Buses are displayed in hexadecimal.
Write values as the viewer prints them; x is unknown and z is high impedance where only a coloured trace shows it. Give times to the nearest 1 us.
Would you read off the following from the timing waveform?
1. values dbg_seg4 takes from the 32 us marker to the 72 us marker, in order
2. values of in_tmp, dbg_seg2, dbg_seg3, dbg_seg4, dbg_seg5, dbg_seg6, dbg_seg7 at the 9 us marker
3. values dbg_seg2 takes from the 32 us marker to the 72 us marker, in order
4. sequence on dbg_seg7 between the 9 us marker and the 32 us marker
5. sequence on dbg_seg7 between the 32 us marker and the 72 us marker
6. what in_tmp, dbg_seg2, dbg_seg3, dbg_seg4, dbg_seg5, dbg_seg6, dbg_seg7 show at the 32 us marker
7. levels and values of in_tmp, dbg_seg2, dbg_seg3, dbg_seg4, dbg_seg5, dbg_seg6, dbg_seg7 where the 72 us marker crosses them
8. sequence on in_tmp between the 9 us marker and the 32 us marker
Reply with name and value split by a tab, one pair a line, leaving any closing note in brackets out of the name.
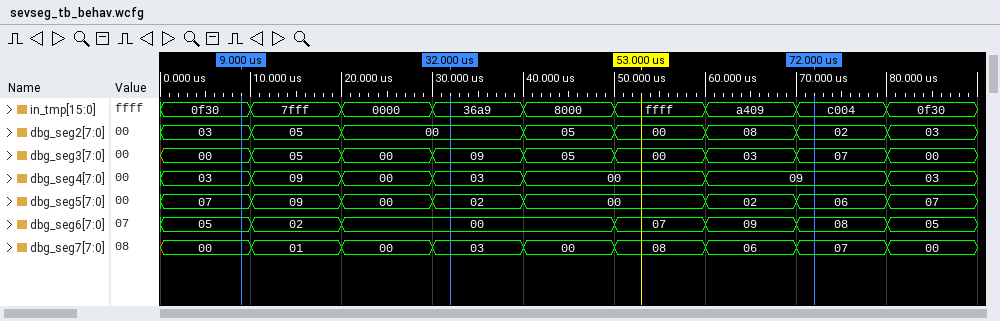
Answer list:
values dbg_seg4 takes from the 32 us marker to the 72 us marker, in order	03, 00, 09
values of in_tmp, dbg_seg2, dbg_seg3, dbg_seg4, dbg_seg5, dbg_seg6, dbg_seg7 at the 9 us marker	in_tmp=0f30, dbg_seg2=03, dbg_seg3=00, dbg_seg4=03, dbg_seg5=07, dbg_seg6=05, dbg_seg7=00
values dbg_seg2 takes from the 32 us marker to the 72 us marker, in order	00, 05, 00, 08, 02
sequence on dbg_seg7 between the 9 us marker and the 32 us marker	00, 01, 00, 03
sequence on dbg_seg7 between the 32 us marker and the 72 us marker	03, 00, 08, 06, 07
what in_tmp, dbg_seg2, dbg_seg3, dbg_seg4, dbg_seg5, dbg_seg6, dbg_seg7 show at the 32 us marker	in_tmp=36a9, dbg_seg2=00, dbg_seg3=09, dbg_seg4=03, dbg_seg5=02, dbg_seg6=00, dbg_seg7=03
levels and values of in_tmp, dbg_seg2, dbg_seg3, dbg_seg4, dbg_seg5, dbg_seg6, dbg_seg7 where the 72 us marker crosses them	in_tmp=c004, dbg_seg2=02, dbg_seg3=07, dbg_seg4=09, dbg_seg5=06, dbg_seg6=08, dbg_seg7=07
sequence on in_tmp between the 9 us marker and the 32 us marker	0f30, 7fff, 0000, 36a9
